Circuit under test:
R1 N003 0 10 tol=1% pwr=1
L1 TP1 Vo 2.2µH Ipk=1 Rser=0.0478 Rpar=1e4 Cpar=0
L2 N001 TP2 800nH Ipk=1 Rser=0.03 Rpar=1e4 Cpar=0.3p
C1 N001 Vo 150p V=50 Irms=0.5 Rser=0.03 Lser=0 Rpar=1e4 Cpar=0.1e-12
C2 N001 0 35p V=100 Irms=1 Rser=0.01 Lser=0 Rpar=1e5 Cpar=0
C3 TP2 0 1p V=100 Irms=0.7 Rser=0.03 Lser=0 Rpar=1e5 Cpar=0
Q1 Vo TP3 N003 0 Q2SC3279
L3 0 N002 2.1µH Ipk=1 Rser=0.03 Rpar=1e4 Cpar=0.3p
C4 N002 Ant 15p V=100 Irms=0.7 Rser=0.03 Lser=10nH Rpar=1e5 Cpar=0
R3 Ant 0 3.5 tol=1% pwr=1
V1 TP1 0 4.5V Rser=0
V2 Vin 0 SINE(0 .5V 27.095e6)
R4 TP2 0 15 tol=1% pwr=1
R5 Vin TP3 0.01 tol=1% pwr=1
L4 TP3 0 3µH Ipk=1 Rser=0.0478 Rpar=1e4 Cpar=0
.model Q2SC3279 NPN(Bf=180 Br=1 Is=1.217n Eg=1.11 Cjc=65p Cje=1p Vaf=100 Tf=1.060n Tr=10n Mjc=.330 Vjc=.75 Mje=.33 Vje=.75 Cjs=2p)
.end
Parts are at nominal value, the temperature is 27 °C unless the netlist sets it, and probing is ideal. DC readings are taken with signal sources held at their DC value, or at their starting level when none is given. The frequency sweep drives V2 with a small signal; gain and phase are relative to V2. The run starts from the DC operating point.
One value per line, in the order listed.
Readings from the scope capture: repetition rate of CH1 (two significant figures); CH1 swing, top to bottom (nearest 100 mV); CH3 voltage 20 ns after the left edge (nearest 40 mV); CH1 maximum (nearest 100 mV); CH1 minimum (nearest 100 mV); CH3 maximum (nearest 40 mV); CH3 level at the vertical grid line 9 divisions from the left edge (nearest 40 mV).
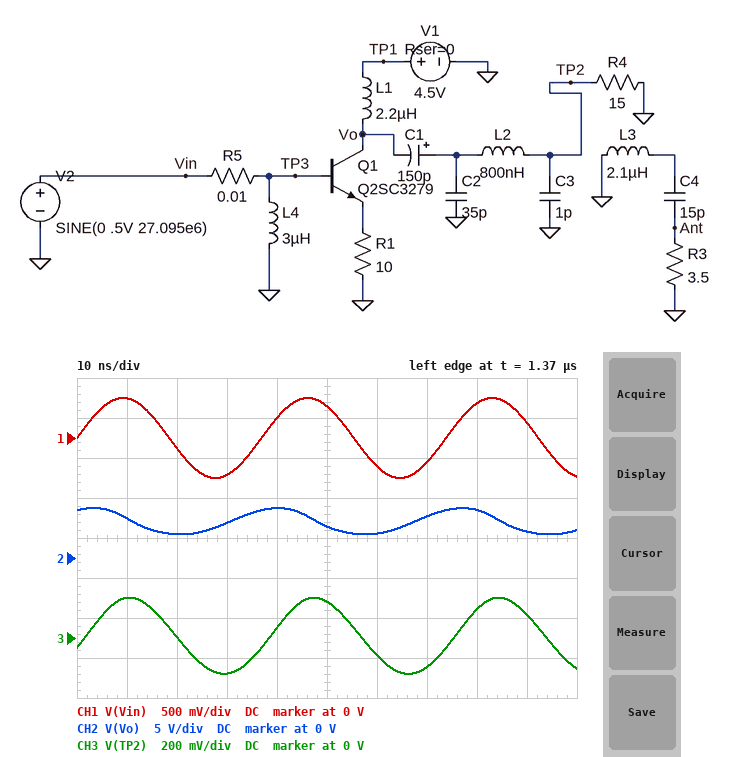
27 MHz
1.0 V
0 V
500 mV
-500 mV
200 mV
120 mV
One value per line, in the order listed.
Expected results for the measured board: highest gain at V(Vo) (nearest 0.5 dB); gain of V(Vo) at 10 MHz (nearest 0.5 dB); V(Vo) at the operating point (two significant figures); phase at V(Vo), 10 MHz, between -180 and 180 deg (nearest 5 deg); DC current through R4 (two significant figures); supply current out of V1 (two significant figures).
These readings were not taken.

11.5 dB
-16.5 dB
4.5 V
30 deg
450 µA
450 µA
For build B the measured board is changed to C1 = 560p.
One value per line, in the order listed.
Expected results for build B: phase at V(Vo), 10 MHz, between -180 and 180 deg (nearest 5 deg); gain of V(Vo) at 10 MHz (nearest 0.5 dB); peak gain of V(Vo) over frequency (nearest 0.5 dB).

150 deg
-24.0 dB
12.5 dB
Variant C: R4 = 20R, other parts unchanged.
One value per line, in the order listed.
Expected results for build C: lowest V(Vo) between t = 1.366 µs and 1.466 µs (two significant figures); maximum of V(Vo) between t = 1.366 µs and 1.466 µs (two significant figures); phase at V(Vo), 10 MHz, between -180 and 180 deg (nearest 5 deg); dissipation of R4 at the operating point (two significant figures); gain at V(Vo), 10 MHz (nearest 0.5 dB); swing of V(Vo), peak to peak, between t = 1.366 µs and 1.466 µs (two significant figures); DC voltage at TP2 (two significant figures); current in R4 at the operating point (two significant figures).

3.1 V
6.1 V
40 deg
4.0 µW
-16.0 dB
3.0 V
9.0 mV
450 µA
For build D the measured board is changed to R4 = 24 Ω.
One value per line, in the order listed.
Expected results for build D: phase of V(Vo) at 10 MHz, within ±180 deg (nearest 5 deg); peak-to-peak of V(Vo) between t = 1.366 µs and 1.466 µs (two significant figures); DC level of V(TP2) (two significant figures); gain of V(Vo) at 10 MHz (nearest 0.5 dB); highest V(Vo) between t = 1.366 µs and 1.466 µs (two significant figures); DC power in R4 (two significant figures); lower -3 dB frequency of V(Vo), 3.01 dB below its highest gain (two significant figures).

45 deg
2.8 V
11 mV
-15.5 dB
6.0 V
4.8 µW
23 MHz
